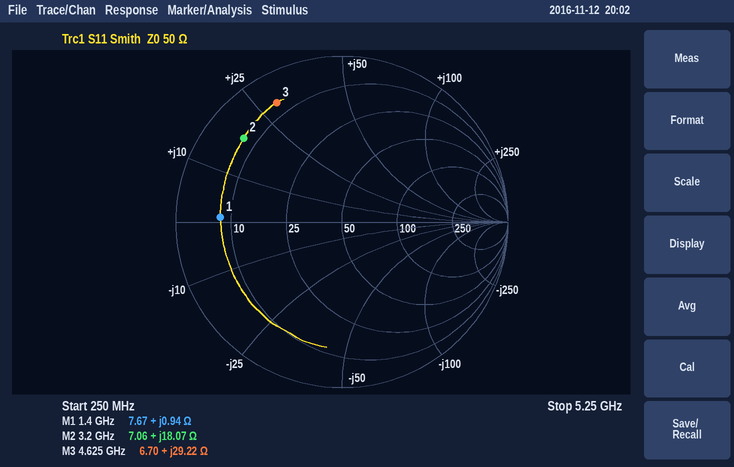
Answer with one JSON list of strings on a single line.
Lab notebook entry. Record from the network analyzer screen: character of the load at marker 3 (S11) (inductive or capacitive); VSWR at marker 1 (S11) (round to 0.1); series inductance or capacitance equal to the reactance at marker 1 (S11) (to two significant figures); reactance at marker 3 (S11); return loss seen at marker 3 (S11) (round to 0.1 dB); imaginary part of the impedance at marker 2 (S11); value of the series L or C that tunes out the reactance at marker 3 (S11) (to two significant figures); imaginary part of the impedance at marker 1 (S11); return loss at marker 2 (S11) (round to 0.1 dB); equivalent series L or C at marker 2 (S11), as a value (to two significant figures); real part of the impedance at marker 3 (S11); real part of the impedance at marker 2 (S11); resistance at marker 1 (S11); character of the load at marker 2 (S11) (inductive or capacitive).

["inductive", "6.5", "110 pH", "+29.22 Ω", "1.7 dB", "+18.07 Ω", "1.2 pF", "+0.94 Ω", "2.2 dB", "900 pH", "6.70 Ω", "7.06 Ω", "7.67 Ω", "inductive"]
